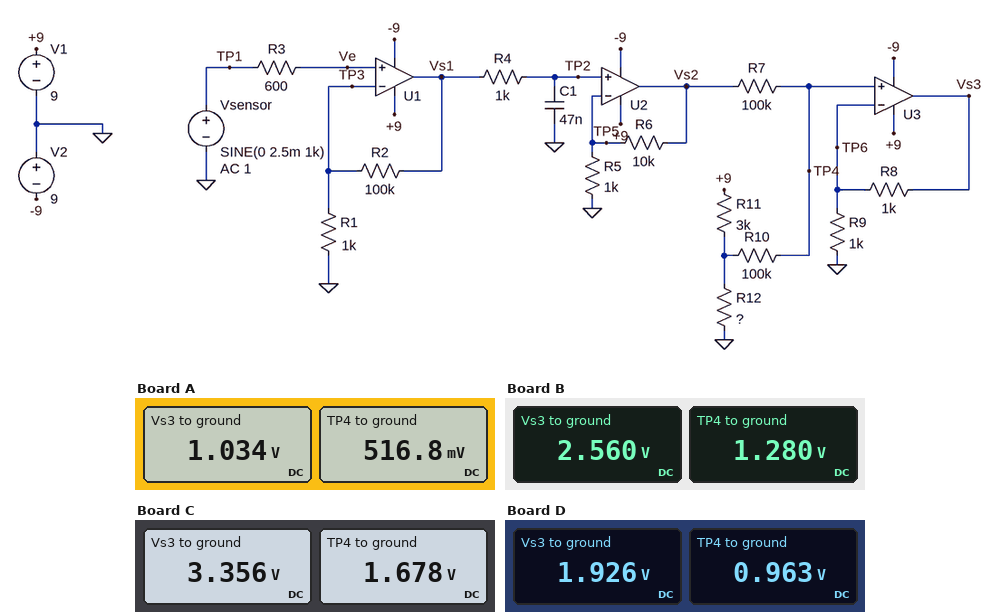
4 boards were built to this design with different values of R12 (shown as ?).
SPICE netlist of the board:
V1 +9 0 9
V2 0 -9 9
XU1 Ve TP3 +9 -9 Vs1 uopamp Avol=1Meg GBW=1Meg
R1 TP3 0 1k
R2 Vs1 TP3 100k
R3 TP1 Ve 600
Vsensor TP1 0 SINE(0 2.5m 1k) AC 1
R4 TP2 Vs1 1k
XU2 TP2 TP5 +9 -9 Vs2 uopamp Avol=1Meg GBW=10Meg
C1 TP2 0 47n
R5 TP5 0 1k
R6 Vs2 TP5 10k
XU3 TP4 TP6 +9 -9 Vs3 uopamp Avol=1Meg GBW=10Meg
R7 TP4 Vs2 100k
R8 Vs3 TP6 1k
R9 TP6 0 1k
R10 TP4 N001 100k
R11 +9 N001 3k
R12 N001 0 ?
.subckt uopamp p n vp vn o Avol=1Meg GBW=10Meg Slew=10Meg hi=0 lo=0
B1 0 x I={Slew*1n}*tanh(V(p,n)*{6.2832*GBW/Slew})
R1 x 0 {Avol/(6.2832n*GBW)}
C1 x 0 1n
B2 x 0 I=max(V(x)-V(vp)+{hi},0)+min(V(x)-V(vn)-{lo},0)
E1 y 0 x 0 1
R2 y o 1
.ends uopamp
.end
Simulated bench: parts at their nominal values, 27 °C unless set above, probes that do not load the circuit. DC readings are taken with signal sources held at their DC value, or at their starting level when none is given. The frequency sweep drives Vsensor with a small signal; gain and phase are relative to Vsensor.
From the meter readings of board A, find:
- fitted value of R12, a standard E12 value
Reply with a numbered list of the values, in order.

1. 390 Ω
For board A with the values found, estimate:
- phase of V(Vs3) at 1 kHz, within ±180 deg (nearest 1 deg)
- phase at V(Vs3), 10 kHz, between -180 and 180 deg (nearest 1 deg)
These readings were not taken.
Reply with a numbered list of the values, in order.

1. -22 deg
2. -117 deg
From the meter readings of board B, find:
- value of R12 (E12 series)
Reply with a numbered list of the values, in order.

1. 1.2 kΩ
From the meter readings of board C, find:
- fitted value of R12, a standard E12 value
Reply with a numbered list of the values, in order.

1. 1.8 kΩ
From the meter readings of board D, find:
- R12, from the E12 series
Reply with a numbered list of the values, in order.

1. 820 Ω
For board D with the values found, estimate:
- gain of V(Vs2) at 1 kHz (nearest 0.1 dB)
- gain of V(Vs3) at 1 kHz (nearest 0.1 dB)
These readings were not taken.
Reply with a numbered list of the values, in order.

1. 60.5 dB
2. 60.5 dB
